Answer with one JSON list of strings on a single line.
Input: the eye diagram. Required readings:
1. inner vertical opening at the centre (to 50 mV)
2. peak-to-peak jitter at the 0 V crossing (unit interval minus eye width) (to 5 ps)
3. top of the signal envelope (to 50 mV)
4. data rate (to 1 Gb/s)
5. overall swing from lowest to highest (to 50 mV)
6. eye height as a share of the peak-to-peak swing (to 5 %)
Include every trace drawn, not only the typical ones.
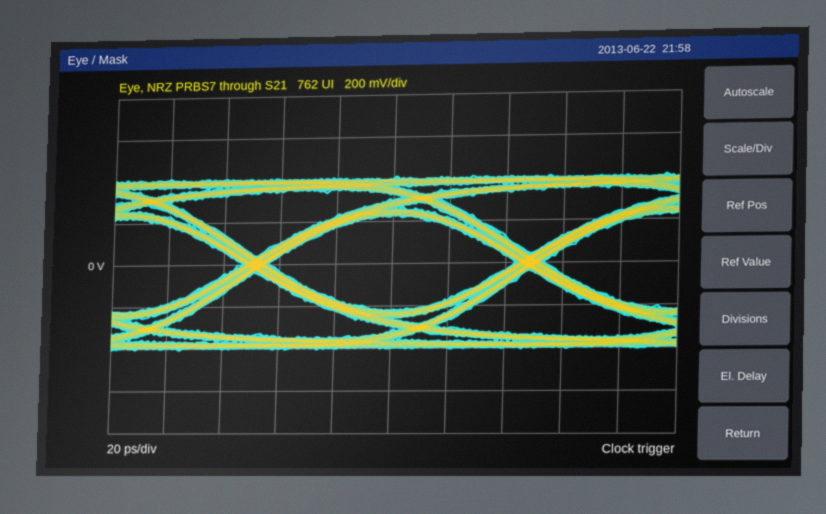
["450 mV", "10 ps", "400 mV", "10 Gb/s", "800 mV", "55 %"]
